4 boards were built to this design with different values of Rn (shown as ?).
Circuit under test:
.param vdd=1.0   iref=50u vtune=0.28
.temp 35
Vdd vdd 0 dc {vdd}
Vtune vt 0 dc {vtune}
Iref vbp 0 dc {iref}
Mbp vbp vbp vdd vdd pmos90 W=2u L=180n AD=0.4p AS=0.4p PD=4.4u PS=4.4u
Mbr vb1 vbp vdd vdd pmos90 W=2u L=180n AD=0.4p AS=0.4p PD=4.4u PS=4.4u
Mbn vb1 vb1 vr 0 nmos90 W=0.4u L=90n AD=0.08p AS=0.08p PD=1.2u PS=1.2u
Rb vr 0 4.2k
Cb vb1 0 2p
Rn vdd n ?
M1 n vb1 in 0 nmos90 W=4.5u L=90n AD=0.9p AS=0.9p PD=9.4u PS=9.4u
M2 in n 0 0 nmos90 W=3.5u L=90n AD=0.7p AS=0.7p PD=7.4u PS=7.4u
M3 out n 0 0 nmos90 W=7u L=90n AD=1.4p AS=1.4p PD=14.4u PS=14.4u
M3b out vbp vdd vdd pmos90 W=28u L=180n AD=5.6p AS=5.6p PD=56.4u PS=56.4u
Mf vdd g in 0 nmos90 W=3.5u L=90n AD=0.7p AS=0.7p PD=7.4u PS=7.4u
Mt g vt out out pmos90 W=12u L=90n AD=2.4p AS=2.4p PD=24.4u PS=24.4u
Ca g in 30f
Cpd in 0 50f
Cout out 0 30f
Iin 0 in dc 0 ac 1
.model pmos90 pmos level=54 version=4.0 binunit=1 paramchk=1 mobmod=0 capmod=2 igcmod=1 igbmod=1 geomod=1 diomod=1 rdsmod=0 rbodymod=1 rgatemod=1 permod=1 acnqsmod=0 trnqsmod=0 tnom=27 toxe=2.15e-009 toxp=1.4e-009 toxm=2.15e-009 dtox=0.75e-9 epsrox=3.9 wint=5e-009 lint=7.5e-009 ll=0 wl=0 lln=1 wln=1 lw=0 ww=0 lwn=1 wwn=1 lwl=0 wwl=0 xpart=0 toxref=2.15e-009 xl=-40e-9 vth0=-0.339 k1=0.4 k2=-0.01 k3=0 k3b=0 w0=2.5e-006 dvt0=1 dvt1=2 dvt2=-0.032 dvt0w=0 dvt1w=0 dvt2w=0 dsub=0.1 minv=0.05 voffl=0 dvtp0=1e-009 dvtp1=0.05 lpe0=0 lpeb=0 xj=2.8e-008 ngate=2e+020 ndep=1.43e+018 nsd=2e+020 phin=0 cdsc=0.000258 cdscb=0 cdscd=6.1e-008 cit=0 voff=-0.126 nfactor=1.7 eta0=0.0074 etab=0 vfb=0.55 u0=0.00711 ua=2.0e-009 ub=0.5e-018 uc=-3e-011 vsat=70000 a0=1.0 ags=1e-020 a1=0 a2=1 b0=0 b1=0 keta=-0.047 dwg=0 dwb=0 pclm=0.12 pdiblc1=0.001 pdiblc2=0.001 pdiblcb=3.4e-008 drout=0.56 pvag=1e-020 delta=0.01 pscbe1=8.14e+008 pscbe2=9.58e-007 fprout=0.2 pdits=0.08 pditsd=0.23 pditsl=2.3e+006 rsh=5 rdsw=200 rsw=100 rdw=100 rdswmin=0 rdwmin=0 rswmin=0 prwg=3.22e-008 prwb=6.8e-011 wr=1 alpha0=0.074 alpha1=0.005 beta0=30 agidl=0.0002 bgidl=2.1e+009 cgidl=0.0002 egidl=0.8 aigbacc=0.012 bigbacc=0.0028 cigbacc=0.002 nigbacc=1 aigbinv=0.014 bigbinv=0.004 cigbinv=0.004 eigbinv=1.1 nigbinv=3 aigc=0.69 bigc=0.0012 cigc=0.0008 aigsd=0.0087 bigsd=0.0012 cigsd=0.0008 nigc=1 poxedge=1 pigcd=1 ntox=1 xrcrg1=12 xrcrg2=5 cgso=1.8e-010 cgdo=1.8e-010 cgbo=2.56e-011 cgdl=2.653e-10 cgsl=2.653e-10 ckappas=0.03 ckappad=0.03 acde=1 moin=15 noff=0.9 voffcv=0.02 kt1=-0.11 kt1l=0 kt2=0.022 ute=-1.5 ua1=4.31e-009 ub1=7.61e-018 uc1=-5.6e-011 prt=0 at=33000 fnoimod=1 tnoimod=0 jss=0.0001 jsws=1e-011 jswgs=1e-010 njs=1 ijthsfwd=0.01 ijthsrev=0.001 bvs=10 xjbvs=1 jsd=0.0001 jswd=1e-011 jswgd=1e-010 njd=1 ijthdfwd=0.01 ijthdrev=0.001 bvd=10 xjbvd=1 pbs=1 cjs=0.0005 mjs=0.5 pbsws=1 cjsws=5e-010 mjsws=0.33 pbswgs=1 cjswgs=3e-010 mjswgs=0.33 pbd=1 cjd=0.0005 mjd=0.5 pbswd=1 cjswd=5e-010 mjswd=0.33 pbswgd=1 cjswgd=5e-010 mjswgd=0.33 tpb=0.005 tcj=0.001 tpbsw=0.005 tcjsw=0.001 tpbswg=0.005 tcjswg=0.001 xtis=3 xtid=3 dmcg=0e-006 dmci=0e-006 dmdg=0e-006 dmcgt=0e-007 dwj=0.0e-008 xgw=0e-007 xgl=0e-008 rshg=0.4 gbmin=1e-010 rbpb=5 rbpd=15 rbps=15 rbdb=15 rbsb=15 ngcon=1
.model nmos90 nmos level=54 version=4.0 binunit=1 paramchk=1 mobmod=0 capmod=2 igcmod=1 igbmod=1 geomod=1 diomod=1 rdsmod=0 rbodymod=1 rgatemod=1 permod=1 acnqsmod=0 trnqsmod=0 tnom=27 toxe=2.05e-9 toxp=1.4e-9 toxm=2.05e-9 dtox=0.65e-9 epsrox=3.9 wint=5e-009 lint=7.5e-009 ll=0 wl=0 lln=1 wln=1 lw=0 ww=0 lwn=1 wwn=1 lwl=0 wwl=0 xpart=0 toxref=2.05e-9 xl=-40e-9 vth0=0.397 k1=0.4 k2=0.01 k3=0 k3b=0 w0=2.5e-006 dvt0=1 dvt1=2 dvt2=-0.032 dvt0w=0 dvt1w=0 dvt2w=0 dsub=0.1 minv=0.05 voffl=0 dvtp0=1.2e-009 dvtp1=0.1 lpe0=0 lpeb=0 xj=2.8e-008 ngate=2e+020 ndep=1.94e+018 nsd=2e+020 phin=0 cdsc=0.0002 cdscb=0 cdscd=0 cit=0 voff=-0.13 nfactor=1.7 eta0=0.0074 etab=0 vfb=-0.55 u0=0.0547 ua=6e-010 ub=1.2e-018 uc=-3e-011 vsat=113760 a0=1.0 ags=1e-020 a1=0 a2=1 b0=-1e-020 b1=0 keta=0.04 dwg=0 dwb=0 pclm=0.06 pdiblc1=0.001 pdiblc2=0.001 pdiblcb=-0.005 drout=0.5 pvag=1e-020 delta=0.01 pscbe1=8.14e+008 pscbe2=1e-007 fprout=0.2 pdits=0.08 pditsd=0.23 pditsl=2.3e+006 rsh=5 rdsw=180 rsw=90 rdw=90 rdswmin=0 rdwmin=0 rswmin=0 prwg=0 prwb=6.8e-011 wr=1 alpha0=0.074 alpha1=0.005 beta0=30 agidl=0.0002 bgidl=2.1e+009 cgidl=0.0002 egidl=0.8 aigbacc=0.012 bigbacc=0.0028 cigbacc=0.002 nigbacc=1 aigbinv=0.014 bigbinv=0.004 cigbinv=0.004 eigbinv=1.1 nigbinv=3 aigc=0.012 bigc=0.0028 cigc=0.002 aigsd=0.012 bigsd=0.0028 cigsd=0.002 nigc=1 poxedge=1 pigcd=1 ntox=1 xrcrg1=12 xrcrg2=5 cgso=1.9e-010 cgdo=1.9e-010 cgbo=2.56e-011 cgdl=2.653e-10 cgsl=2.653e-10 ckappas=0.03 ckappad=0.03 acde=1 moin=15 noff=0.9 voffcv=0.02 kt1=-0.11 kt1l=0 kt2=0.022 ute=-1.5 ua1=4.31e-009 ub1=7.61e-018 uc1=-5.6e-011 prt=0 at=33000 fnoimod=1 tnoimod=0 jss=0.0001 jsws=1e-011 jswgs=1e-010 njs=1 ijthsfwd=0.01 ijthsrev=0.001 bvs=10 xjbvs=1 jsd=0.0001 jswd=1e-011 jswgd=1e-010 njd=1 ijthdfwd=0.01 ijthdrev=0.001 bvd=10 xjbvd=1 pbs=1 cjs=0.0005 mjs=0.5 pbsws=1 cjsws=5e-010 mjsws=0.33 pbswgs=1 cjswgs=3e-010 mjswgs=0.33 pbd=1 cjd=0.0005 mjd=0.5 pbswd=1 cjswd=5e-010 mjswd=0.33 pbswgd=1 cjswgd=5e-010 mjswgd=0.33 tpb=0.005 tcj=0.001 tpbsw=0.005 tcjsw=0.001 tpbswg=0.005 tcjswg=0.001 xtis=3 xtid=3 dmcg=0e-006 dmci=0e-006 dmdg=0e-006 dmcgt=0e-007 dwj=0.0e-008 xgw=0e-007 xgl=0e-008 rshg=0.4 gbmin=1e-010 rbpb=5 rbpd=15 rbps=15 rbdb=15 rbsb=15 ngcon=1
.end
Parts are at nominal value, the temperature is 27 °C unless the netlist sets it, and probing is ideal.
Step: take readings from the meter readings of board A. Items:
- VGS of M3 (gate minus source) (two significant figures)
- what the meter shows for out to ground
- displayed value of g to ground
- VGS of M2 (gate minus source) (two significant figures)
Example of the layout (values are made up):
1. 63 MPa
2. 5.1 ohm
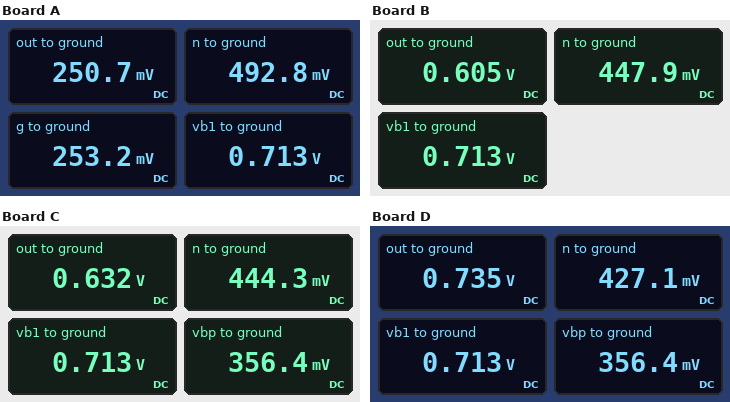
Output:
1. 490 mV
2. 250.7 mV
3. 253.2 mV
4. 490 mV
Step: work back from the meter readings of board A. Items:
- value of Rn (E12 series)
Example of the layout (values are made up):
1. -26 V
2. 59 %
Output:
1. 1.5 kΩ
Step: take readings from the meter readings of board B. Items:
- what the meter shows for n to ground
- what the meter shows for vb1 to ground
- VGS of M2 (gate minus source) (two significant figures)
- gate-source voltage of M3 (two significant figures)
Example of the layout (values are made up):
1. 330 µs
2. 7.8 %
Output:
1. 447.9 mV
2. 0.713 V
3. 450 mV
4. 450 mV
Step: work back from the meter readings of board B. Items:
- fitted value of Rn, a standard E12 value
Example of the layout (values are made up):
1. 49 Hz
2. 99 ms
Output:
1. 3.3 kΩ
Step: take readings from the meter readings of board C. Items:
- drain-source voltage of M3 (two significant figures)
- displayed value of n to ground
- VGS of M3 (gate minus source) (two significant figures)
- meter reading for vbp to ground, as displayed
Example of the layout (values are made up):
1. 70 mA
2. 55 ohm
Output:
1. 630 mV
2. 444.3 mV
3. 440 mV
4. 356.4 mV
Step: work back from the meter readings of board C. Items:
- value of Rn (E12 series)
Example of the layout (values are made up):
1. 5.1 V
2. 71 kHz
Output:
1. 3.9 kΩ
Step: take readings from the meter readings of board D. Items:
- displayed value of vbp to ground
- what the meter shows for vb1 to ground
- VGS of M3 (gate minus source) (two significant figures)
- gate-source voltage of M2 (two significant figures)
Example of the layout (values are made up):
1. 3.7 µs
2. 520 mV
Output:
1. 356.4 mV
2. 0.713 V
3. 430 mV
4. 430 mV
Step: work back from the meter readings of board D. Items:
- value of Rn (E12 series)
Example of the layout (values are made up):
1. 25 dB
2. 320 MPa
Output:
1. 12 kΩ
